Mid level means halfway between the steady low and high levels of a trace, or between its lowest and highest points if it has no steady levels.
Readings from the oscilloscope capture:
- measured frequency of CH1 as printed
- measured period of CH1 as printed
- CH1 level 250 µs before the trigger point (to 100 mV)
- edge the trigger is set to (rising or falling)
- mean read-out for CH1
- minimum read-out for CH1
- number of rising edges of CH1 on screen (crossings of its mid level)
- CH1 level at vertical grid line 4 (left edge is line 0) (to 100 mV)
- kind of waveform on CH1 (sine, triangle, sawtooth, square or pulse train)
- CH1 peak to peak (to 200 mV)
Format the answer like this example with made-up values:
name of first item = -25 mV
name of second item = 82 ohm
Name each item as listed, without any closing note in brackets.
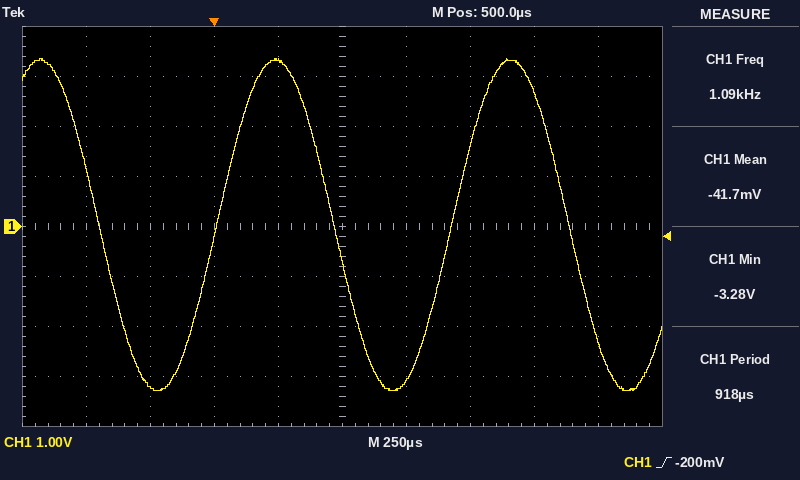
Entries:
measured frequency of CH1 as printed = 1.09 kHz
measured period of CH1 as printed = 918 µs
CH1 level 250 µs before the trigger point = -3.2 V
edge the trigger is set to = rising
mean read-out for CH1 = -41.7 mV
minimum read-out for CH1 = -3.28 V
number of rising edges of CH1 on screen = 2
CH1 level at vertical grid line 4 (left edge is line 0) = 3.3 V
kind of waveform on CH1 = sine
CH1 peak to peak = 6.6 V
